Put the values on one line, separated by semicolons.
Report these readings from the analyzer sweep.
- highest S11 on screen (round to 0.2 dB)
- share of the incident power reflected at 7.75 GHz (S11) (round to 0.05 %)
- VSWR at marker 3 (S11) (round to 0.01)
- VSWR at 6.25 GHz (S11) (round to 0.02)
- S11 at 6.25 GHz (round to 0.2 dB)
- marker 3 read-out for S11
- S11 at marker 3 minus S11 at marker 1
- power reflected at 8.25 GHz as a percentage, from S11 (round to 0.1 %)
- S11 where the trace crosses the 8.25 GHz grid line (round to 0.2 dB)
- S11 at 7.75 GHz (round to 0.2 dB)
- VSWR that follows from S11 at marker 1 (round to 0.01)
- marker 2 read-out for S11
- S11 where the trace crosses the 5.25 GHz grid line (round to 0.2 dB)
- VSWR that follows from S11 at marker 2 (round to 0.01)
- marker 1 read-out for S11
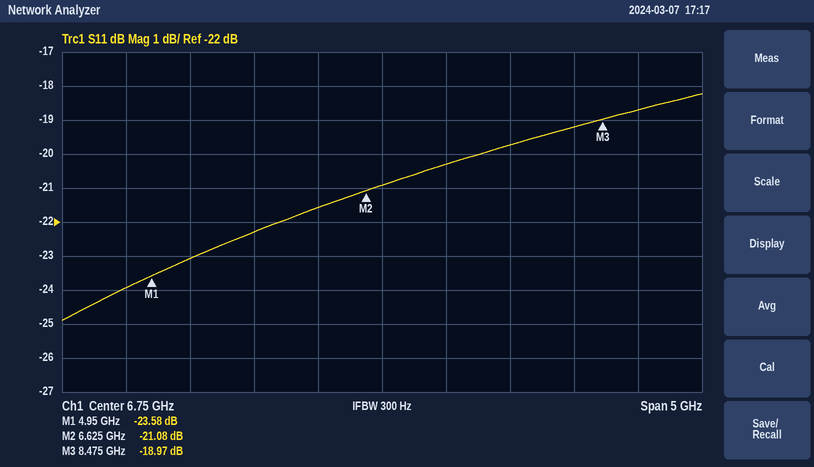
-18.2 dB; 1.05 %; 1.25; 1.18; -21.6 dB; -18.97 dB; 4.61 dB; 1.2 %; -19.2 dB; -19.8 dB; 1.14; -21.08 dB; -23.0 dB; 1.19; -23.58 dB
